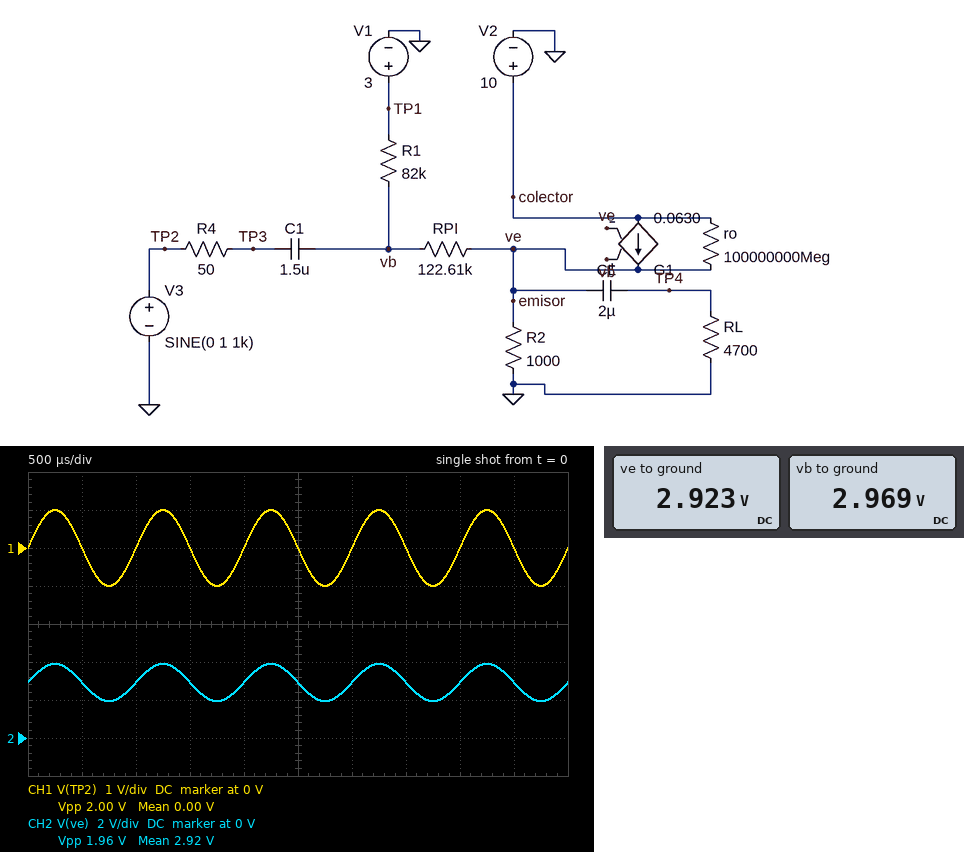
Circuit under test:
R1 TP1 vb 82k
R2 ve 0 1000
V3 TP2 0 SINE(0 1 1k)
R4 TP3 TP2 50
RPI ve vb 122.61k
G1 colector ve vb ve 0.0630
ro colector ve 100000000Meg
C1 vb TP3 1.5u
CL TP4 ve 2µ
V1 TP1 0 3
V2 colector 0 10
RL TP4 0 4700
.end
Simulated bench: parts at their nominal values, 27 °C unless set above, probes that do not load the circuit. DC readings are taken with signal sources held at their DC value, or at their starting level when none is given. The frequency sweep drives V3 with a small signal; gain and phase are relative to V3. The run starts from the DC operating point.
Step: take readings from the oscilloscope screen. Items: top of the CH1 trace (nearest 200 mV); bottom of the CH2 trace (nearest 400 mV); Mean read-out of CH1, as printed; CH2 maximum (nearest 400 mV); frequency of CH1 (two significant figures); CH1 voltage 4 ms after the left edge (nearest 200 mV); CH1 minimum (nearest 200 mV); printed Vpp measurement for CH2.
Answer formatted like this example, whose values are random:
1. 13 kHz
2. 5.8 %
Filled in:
1. 1.0 V
2. 2.0 V
3. 0.00 V
4. 4.0 V
5. 1.0 kHz
6. 0 V
7. -1.0 V
8. 1.96 V
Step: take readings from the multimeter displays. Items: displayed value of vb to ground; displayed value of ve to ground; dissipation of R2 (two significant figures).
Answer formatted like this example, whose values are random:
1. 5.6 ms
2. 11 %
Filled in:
1. 2.969 V
2. 2.923 V
3. 8.5 mW
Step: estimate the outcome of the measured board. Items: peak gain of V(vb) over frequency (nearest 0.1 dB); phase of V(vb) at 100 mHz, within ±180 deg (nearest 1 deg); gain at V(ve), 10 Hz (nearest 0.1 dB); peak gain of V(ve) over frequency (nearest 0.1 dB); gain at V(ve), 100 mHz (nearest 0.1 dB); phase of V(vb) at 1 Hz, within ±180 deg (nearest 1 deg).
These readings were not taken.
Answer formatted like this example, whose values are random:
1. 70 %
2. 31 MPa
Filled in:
1. 0 dB
2. 86 deg
3. -0.2 dB
4. -0.2 dB
5. -22.5 dB
6. 53 deg
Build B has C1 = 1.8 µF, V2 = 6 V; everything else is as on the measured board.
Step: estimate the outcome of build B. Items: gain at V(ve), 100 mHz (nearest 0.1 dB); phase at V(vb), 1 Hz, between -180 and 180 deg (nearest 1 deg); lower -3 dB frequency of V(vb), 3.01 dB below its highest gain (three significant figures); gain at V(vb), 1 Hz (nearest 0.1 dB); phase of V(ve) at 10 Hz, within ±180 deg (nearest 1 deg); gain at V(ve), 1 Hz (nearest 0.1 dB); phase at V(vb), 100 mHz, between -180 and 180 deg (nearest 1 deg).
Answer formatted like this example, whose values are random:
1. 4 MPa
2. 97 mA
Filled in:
1. -20.9 dB
2. 47 deg
3. 1.09 Hz
4. -3.4 dB
5. 6 deg
6. -3.5 dB
7. 85 deg
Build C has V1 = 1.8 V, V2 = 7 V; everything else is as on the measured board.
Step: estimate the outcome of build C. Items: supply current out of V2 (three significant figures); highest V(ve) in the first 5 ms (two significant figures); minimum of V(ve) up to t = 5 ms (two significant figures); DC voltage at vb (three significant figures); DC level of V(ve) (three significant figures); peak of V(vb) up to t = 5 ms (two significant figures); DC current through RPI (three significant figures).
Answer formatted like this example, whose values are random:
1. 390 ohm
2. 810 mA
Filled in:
1. 1.75 mA
2. 2.7 V
3. 770 mV
4. 1.78 V
5. 1.75 V
6. 2.8 V
7. 227 nA
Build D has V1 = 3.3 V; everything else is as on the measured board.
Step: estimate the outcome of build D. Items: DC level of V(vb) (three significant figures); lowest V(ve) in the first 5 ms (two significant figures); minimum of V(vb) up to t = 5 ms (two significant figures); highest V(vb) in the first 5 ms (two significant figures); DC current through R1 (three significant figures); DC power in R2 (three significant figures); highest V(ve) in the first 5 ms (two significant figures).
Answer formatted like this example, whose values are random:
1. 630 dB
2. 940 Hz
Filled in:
1. 3.27 V
2. 2.2 V
3. 2.3 V
4. 4.3 V
5. 416 nA
6. 10.3 mW
7. 4.2 V
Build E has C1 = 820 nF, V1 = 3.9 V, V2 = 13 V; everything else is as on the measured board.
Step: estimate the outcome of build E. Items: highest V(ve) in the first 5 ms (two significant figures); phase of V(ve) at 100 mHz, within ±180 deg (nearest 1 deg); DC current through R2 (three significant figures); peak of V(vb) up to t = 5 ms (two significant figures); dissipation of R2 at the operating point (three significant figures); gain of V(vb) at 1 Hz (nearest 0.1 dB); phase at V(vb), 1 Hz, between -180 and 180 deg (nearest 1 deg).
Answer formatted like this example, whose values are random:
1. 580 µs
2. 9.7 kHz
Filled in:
1. 4.8 V
2. 88 deg
3. 3.80 mA
4. 4.9 V
5. 14.4 mW
6. -8.3 dB
7. 67 deg
